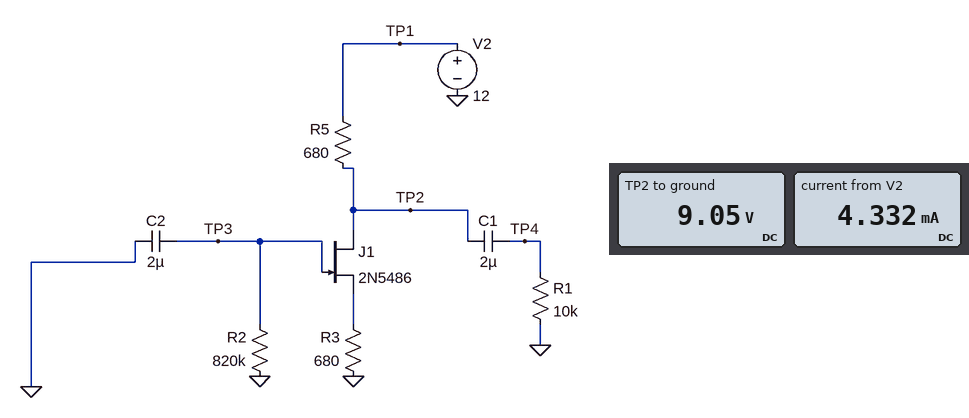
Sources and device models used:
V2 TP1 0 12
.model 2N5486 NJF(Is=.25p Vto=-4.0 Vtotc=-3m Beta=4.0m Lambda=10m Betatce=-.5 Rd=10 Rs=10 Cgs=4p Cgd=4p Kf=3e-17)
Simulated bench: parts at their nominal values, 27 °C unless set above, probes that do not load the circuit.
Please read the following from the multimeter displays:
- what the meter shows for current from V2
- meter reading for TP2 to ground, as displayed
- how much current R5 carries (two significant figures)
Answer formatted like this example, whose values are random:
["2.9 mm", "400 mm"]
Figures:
["4.332 mA", "9.05 V", "4.3 mA"]
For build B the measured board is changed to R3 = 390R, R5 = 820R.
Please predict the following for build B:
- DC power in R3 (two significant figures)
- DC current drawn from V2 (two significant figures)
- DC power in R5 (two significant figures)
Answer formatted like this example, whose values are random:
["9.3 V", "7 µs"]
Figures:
["18 mW", "6.8 mA", "38 mW"]
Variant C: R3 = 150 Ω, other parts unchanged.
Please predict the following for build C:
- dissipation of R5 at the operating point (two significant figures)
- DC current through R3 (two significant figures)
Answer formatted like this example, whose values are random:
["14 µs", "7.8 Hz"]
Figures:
["110 mW", "13 mA"]
